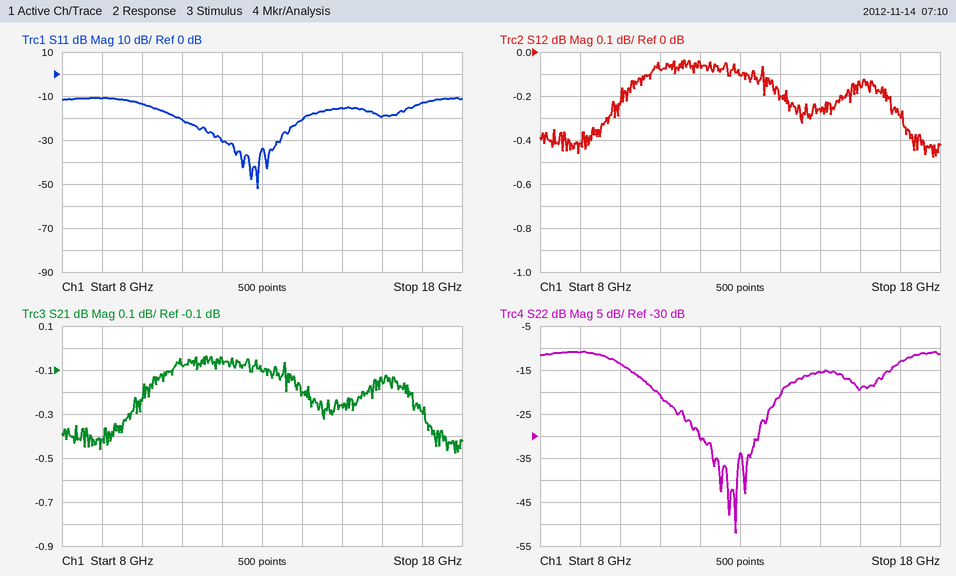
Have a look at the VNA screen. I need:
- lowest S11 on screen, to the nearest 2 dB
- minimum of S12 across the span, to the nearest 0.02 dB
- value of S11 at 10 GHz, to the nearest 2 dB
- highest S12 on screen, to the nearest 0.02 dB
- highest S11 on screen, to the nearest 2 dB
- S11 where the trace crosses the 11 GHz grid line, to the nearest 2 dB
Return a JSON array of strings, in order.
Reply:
["-52 dB", "-0.48 dB", "-14 dB", "-0.04 dB", "-10 dB", "-20 dB"]
